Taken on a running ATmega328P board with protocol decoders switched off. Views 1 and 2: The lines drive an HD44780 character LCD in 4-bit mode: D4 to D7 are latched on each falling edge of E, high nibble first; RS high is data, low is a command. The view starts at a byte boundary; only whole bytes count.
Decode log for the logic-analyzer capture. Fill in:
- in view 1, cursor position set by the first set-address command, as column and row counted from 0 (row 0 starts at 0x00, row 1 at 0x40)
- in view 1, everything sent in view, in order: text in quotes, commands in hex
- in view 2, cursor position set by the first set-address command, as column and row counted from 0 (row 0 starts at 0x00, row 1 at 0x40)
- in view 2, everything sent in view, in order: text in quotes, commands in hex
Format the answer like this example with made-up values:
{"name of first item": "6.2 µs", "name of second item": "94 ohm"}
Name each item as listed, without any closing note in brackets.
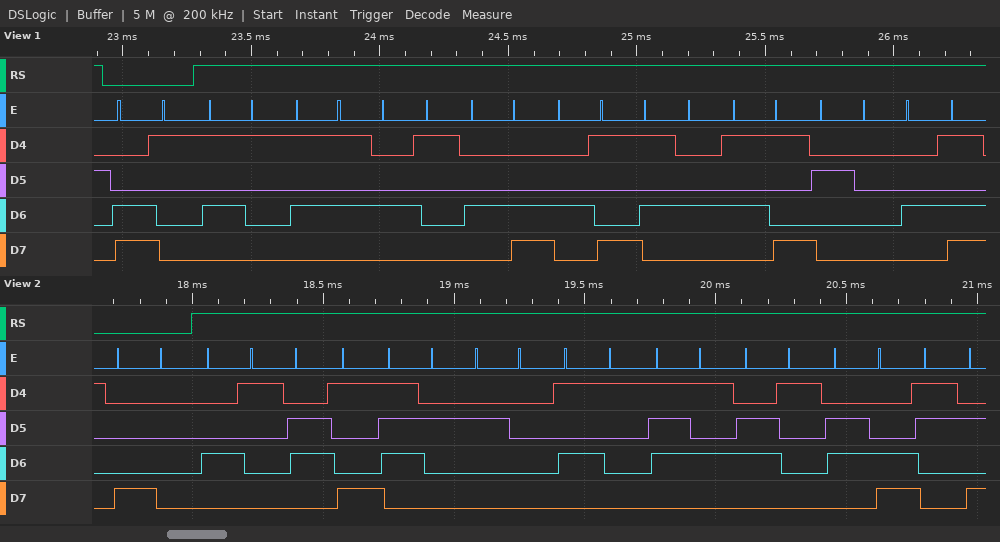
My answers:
{"in view 1, cursor position set by the first set-address command, as column and row counted from 0": "column 1, row 1", "in view 1, everything sent in view, in order: text in quotes, commands in hex": "0xC1 \"QUALITY M\"", "in view 2, cursor position set by the first set-address command, as column and row counted from 0": "column 0, row 0", "in view 2, everything sent in view, in order: text in quotes, commands in hex": "0x80 \"Air Qual:\""}
